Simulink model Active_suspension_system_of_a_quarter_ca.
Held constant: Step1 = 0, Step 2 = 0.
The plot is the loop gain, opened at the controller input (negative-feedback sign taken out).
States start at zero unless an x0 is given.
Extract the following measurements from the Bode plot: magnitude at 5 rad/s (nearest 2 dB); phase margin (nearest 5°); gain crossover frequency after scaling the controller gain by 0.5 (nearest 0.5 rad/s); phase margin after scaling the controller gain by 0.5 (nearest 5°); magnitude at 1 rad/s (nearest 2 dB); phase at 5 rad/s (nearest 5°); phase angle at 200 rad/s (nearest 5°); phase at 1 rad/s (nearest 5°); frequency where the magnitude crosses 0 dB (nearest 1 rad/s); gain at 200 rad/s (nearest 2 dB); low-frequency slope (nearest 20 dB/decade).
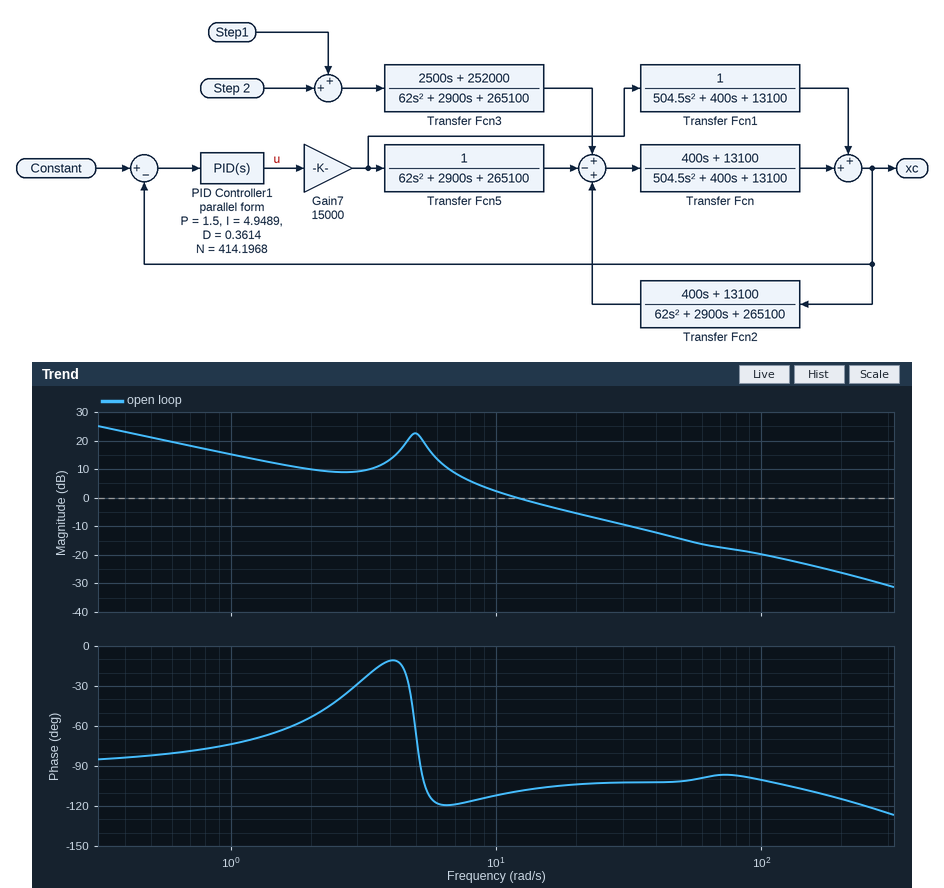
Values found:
22 dB
70°
8.0 rad/s
65°
16 dB
-65°
-115°
-75°
12 rad/s
-26 dB
-20 dB/decade
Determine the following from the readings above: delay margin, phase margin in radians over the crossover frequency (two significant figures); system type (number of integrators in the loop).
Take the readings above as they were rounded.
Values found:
0.10 s
1
